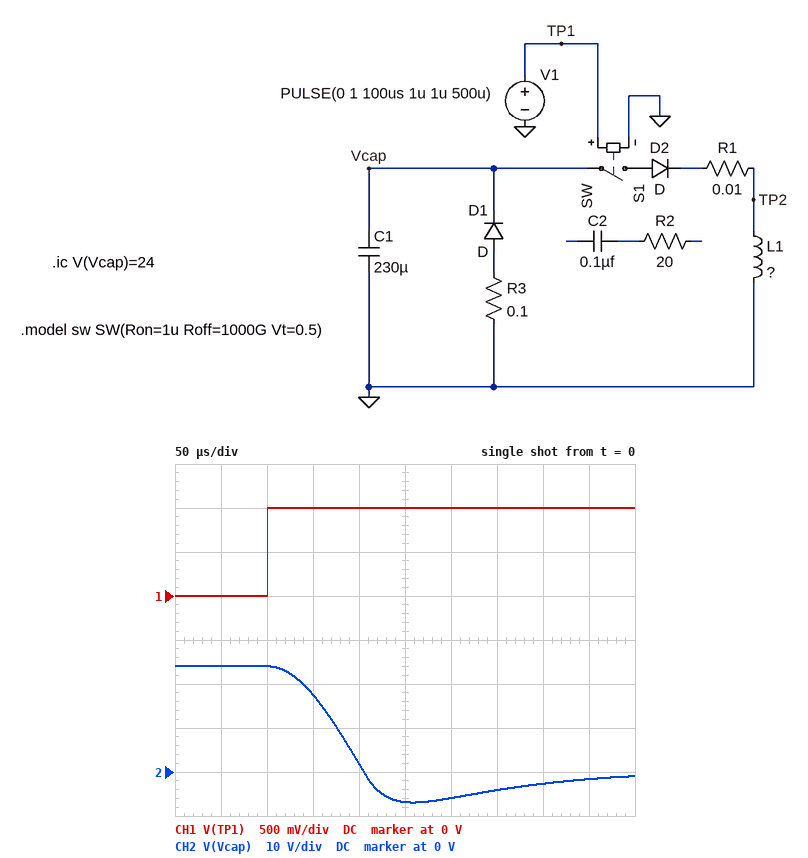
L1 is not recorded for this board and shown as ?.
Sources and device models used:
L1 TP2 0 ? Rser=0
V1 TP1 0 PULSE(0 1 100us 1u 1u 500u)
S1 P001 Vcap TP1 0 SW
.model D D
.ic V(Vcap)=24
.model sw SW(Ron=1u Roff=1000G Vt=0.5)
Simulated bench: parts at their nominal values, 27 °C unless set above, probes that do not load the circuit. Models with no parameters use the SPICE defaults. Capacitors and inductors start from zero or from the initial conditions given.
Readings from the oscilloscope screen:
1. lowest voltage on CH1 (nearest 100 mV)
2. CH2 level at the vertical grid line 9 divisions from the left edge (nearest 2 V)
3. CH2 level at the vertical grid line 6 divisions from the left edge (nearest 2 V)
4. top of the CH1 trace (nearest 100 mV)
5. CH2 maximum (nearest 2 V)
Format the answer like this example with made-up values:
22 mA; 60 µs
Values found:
0 V; -2 V; -6 V; 1.0 V; 24 V
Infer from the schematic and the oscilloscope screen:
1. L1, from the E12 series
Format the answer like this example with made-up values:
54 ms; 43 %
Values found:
18 µH
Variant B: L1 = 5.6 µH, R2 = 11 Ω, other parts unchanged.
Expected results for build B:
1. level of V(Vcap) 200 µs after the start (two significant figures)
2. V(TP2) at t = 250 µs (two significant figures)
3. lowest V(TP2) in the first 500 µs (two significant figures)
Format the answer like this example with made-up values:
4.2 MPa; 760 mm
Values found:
-9.3 V; -4.7 V; -11 V
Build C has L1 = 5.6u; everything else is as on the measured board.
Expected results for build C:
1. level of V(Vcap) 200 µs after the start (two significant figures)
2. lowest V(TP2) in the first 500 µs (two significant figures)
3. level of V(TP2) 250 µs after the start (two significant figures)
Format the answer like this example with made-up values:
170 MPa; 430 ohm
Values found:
-9.3 V; -11 V; -4.7 V
